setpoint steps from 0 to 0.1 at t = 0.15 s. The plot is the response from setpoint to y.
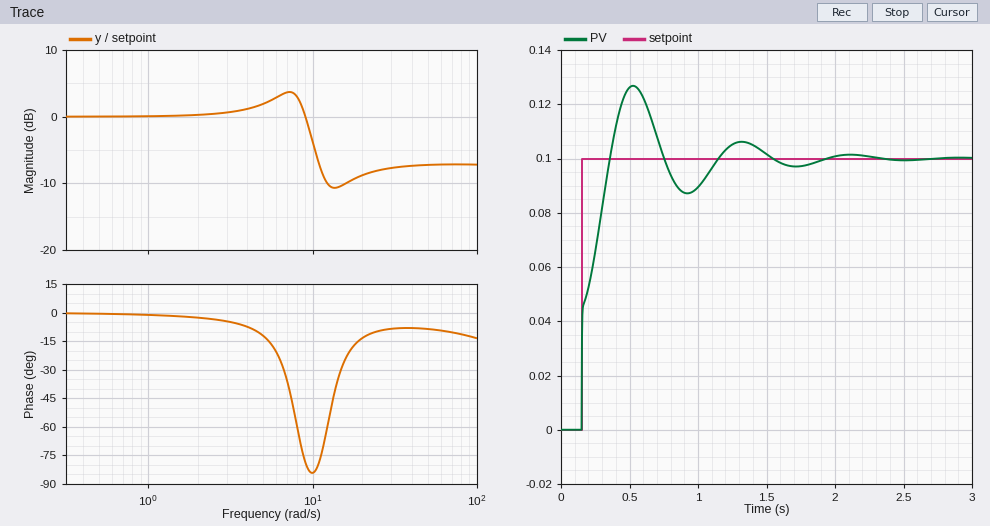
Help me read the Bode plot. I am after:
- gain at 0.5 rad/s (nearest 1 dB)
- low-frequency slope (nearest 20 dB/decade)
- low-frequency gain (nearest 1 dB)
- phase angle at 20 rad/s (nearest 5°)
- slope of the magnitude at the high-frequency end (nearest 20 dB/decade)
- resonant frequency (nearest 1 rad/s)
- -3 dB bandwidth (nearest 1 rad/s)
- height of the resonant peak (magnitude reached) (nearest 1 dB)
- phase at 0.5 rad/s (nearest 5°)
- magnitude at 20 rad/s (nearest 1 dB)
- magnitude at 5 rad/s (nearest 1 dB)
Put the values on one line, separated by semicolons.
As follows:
0 dB; 0 dB/decade; 0 dB; -15°; 0 dB/decade; 7 rad/s; 10 rad/s; 4 dB; 0°; -9 dB; 2 dB
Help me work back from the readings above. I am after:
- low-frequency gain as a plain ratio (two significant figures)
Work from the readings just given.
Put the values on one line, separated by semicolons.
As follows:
1.0
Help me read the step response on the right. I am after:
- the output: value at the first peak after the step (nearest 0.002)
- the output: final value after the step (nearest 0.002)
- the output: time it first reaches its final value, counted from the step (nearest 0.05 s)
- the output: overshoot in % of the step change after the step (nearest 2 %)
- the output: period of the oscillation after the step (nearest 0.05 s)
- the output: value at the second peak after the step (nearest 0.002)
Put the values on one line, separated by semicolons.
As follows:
0.126; 0.100; 0.20 s; 26 %; 0.80 s; 0.106
